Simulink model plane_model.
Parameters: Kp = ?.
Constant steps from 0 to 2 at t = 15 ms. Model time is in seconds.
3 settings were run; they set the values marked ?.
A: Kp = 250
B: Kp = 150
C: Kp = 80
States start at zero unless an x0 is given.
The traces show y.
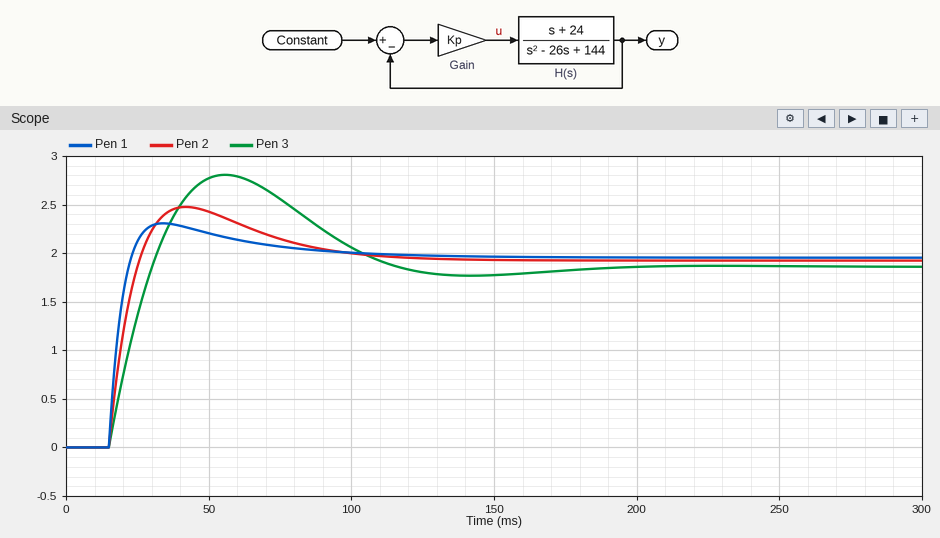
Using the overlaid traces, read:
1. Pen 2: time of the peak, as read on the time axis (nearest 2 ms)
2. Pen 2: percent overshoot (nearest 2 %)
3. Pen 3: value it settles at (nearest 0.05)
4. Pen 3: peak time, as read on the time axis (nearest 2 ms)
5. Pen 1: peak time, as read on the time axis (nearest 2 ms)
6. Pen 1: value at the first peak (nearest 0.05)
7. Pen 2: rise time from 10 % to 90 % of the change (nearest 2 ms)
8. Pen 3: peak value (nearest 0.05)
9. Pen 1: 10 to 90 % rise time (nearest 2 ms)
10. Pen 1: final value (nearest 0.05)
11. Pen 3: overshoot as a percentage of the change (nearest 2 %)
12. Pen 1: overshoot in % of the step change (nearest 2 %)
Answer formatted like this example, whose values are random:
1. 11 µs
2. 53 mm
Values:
1. 42 ms
2. 28 %
3. 1.85
4. 56 ms
5. 34 ms
6. 2.30
7. 8 ms
8. 2.80
9. 6 ms
10. 1.95
11. 50 %
12. 18 %
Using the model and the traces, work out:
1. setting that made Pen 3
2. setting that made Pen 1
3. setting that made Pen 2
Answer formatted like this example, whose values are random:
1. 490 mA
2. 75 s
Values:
1. C
2. A
3. B
